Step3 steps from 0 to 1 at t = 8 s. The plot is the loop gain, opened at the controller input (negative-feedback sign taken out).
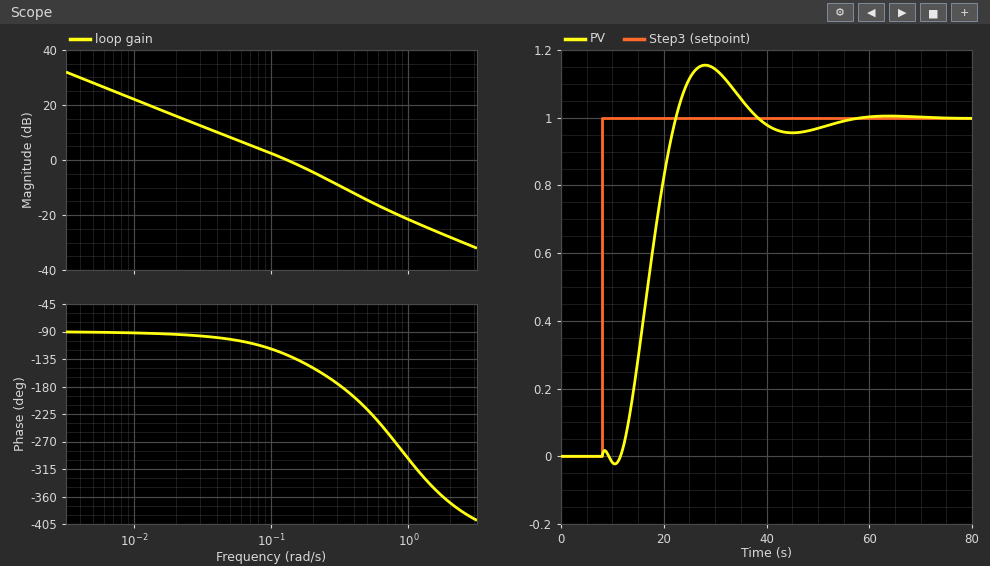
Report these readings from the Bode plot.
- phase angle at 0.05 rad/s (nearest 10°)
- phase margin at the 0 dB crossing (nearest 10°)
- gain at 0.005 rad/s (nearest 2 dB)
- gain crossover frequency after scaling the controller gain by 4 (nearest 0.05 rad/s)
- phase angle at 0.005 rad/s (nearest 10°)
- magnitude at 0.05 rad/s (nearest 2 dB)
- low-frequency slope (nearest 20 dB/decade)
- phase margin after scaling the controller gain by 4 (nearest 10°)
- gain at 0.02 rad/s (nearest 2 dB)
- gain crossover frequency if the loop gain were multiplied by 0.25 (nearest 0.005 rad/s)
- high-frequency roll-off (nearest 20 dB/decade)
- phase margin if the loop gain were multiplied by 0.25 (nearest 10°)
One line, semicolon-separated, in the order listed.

-100°; 50°; 28 dB; 0.40 rad/s; -90°; 8 dB; -20 dB/decade; -20°; 16 dB; 0.030 rad/s; -20 dB/decade; 80°
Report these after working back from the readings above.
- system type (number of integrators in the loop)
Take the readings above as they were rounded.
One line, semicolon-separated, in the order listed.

1
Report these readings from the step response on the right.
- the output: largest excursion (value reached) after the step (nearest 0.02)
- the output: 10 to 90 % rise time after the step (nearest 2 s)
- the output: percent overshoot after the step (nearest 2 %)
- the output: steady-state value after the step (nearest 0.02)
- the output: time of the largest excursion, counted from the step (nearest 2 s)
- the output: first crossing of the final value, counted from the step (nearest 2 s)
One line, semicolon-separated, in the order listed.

1.16; 8 s; 16 %; 1.00; 20 s; 14 s
